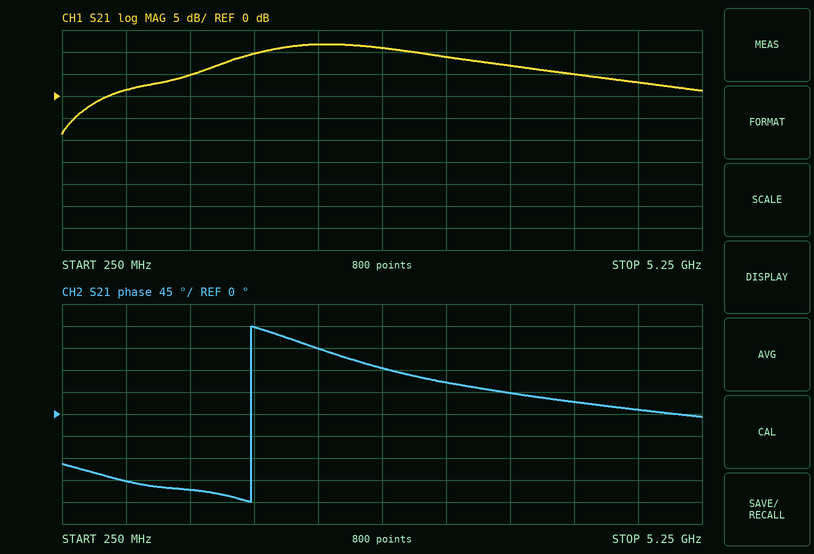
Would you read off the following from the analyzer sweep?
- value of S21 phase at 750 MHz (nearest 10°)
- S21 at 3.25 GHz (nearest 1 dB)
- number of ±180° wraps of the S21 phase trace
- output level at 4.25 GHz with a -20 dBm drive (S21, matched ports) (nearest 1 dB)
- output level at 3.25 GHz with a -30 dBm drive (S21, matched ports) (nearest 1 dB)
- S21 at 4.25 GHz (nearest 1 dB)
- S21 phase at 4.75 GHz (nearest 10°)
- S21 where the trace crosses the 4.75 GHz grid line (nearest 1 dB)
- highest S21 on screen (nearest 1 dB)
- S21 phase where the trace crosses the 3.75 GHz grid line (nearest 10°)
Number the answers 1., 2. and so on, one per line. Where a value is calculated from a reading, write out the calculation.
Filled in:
1. -140°
2. 9 dB
3. 1
4. -20 dBm + (5 dB) = -15 dBm
5. -30 dBm + (9 dB) = -21 dBm
6. 5 dB
7. 10°
8. 3 dB
9. 12 dB
10. 40°
